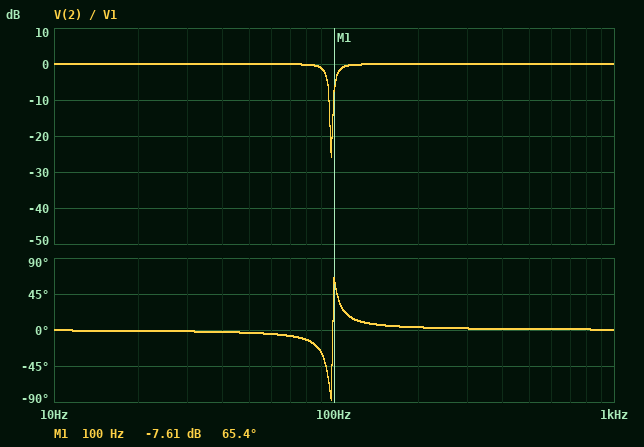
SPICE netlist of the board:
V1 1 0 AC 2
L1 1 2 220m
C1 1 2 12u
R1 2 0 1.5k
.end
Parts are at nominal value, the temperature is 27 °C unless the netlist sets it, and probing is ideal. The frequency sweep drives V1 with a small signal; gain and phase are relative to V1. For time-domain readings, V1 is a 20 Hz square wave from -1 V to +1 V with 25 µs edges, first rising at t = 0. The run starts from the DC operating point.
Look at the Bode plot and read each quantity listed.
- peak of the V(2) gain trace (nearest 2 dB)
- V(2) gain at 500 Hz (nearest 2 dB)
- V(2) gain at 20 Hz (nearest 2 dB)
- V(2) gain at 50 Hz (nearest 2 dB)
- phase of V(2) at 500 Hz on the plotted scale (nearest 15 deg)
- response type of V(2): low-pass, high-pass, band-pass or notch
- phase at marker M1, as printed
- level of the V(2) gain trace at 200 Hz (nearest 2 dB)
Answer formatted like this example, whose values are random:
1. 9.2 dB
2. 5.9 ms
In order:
1. 0 dB
2. 0 dB
3. 0 dB
4. 0 dB
5. 0 deg
6. notch
7. 65.4 deg
8. 0 dB
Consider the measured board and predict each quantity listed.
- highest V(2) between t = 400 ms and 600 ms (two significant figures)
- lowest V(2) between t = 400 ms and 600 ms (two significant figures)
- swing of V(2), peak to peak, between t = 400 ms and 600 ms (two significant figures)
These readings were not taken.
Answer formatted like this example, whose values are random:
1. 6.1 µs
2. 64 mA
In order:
1. 1.3 V
2. -1.3 V
3. 2.5 V
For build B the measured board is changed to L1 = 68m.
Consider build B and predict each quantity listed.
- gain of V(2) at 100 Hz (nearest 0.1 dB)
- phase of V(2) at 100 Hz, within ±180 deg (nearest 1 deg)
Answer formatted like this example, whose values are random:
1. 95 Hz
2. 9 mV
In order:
1. 0 dB
2. -2 deg
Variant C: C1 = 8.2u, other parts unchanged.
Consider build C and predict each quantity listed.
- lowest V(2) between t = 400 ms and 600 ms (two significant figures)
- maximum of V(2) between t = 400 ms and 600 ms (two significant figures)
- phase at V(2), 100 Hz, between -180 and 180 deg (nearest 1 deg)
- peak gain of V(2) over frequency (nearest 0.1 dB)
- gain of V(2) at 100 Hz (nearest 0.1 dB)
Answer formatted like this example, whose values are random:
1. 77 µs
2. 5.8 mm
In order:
1. -1.1 V
2. 1.1 V
3. -18 deg
4. 0 dB
5. -0.4 dB
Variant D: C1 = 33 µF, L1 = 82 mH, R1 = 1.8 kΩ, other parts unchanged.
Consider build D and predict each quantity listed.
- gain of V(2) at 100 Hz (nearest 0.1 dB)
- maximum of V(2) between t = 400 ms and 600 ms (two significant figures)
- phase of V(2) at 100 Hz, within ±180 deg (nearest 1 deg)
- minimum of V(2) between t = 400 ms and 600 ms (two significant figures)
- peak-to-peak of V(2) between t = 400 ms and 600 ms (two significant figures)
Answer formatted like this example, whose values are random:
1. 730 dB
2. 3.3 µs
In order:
1. -0.7 dB
2. 1.1 V
3. 23 deg
4. -1.1 V
5. 2.2 V
